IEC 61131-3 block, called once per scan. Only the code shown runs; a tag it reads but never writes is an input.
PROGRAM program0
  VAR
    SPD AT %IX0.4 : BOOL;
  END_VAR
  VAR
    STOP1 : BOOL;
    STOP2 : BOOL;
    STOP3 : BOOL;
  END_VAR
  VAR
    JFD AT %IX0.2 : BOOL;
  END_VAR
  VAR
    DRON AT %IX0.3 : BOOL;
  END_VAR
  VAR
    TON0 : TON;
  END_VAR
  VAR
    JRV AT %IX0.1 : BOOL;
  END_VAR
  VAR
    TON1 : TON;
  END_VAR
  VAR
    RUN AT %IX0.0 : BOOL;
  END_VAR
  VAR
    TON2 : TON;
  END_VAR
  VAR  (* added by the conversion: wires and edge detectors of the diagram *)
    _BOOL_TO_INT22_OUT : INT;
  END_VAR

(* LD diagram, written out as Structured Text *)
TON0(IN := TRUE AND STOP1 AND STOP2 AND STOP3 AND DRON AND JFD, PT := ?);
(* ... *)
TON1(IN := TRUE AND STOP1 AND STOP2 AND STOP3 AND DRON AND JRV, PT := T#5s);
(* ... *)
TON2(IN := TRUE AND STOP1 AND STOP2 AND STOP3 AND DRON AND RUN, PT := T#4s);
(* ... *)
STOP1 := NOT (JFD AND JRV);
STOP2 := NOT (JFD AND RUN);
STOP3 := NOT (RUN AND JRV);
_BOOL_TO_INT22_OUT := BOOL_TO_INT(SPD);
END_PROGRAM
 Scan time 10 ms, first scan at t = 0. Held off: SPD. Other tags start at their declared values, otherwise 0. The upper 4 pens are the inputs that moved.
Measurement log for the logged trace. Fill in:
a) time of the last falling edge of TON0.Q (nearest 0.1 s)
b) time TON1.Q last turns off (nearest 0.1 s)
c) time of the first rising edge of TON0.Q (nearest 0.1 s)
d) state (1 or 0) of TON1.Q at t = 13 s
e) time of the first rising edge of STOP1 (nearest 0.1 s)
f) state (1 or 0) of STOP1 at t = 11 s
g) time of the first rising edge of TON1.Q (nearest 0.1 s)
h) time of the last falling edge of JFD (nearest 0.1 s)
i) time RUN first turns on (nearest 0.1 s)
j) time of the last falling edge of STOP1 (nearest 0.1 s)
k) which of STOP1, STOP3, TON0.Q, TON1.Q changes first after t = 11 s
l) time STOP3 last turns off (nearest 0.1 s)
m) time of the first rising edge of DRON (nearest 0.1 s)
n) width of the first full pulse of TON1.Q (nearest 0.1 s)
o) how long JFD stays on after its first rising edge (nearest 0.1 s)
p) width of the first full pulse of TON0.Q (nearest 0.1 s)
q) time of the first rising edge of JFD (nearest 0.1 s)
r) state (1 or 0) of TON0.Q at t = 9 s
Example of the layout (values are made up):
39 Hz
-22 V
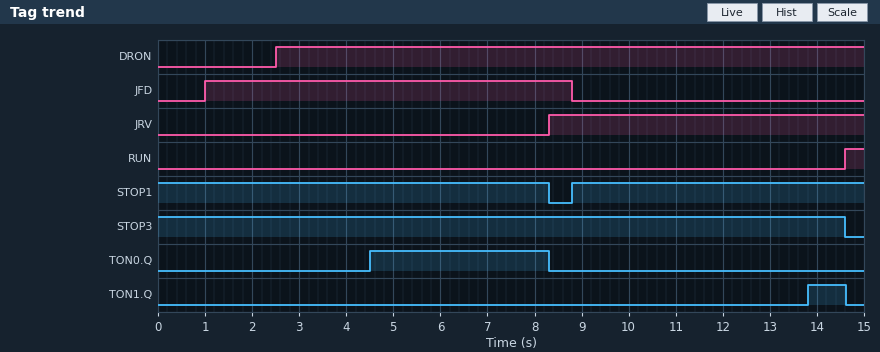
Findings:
8.3 s
14.6 s
4.5 s
0
8.8 s
1
13.8 s
8.8 s
14.6 s
8.3 s
TON1.Q
14.6 s
2.5 s
0.8 s
7.8 s
3.8 s
1.0 s
0
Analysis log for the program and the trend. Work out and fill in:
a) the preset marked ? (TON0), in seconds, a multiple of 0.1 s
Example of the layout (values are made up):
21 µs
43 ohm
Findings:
2.0 s
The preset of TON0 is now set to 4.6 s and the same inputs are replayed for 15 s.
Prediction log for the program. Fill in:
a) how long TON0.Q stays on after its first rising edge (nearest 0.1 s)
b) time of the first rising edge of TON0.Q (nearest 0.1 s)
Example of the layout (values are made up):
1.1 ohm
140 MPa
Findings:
1.2 s
7.1 s
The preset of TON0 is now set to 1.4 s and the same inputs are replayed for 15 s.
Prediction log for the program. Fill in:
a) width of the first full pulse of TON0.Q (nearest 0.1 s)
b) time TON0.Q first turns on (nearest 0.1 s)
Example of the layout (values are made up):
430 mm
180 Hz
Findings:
4.4 s
3.9 s
